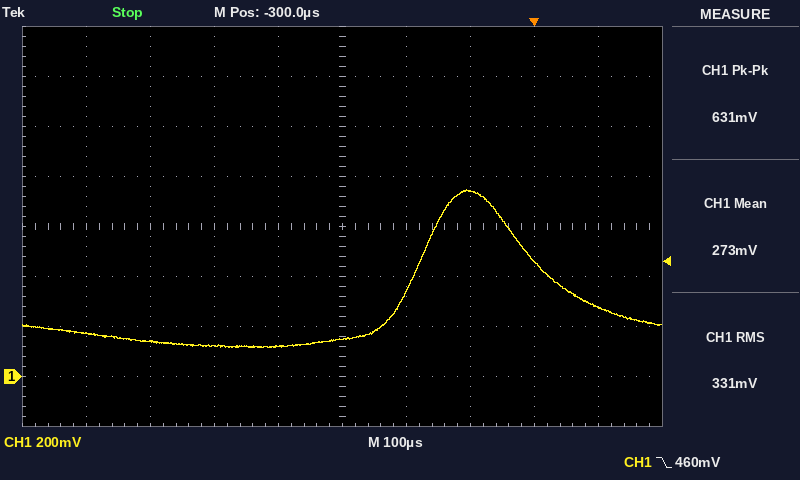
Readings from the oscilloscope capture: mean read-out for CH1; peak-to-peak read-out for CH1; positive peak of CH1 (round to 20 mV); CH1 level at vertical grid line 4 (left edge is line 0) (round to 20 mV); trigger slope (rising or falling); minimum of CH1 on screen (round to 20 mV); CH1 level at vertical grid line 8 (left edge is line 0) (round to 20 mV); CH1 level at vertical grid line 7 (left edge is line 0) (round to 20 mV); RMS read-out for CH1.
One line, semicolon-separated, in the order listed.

273 mV; 631 mV; 740 mV; 120 mV; falling; 120 mV; 460 mV; 740 mV; 331 mV
